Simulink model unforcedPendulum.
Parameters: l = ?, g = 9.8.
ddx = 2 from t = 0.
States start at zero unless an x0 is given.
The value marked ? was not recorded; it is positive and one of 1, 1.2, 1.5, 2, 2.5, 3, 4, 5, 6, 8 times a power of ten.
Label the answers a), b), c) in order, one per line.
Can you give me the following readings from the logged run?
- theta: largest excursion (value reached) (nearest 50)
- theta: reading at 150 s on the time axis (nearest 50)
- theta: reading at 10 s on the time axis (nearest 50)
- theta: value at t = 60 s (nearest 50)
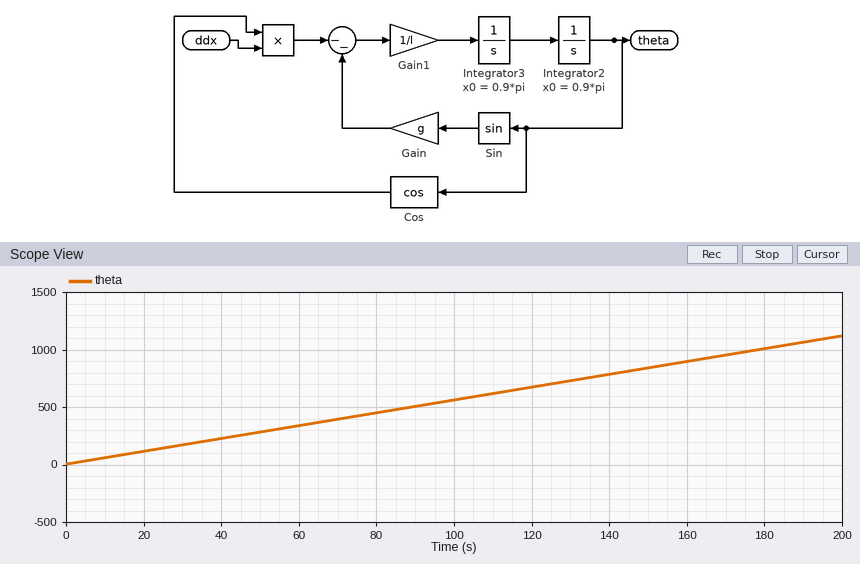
a) 1100
b) 850
c) 50
d) 350
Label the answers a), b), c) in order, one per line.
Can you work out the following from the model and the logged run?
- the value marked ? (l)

a) 0.5
